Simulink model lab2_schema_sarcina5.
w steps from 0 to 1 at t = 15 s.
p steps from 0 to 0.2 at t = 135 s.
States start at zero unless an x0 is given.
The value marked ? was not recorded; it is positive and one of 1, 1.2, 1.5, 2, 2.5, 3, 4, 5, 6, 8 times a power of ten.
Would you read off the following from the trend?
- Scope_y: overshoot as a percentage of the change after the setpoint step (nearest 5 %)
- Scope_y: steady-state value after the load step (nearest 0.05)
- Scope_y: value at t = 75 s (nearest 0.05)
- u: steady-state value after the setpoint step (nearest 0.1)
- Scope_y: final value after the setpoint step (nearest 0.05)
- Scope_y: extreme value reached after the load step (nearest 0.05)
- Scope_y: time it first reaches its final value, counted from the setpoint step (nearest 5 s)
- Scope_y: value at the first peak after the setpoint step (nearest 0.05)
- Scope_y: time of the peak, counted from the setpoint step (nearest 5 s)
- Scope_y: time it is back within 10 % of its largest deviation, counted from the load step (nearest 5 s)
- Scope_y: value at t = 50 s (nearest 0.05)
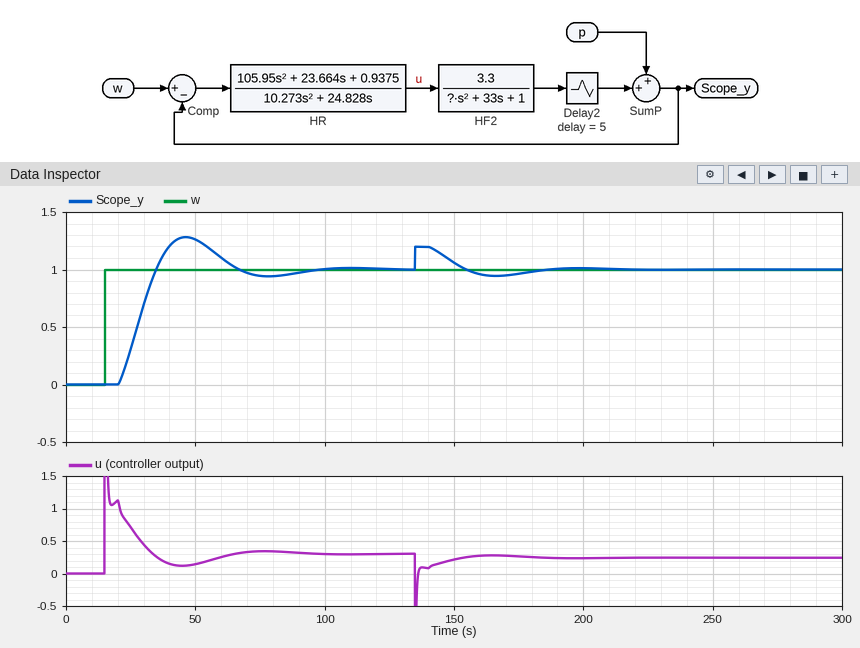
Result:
30 %
1.00
0.95
0.3
1.00
1.20
20 s
1.30
30 s
45 s
1.25
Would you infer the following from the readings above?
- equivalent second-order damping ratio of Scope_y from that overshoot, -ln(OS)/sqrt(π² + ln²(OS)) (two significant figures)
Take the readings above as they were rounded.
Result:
0.36
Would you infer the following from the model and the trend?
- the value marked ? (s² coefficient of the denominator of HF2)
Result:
250
